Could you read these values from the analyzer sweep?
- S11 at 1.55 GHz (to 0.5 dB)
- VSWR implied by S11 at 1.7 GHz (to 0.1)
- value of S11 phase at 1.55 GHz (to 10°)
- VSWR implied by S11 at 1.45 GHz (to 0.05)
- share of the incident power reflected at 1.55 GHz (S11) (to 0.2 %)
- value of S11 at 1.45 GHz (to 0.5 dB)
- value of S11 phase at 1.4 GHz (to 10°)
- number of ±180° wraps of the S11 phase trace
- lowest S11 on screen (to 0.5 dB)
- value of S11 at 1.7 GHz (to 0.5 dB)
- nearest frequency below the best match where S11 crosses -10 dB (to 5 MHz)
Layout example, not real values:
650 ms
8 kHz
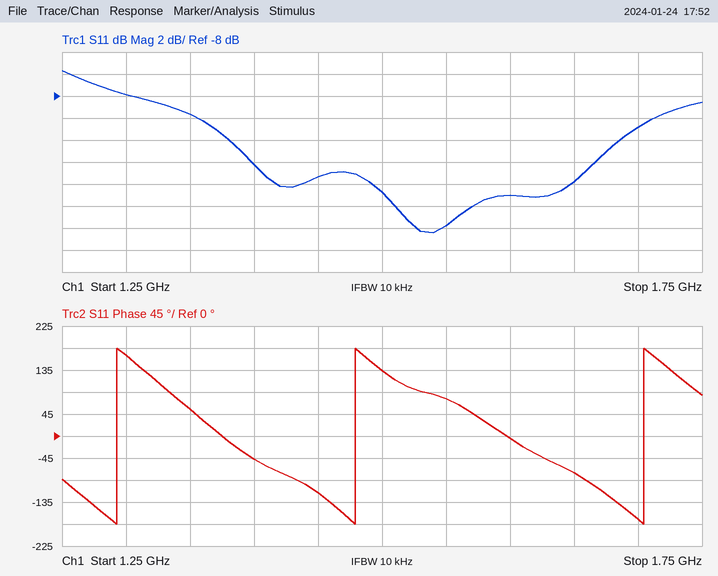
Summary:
-20.0 dB
1.8
80°
1.40
1.0 %
-15.5 dB
-50°
3
-20.5 dB
-11.0 dB
1.355 GHz
